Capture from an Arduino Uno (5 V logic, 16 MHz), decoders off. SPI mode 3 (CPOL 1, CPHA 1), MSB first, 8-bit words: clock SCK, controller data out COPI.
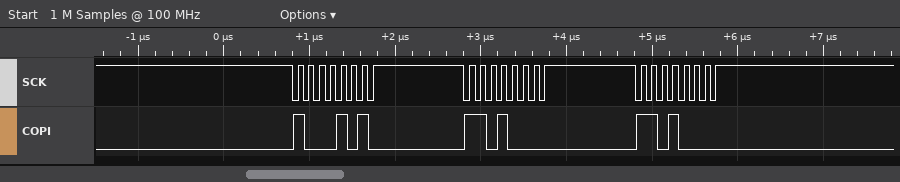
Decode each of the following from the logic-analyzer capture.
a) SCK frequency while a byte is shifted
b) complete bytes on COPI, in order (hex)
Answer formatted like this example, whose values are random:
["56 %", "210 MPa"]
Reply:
["8 MHz", "0x8A 0xD0 0xD0"]
